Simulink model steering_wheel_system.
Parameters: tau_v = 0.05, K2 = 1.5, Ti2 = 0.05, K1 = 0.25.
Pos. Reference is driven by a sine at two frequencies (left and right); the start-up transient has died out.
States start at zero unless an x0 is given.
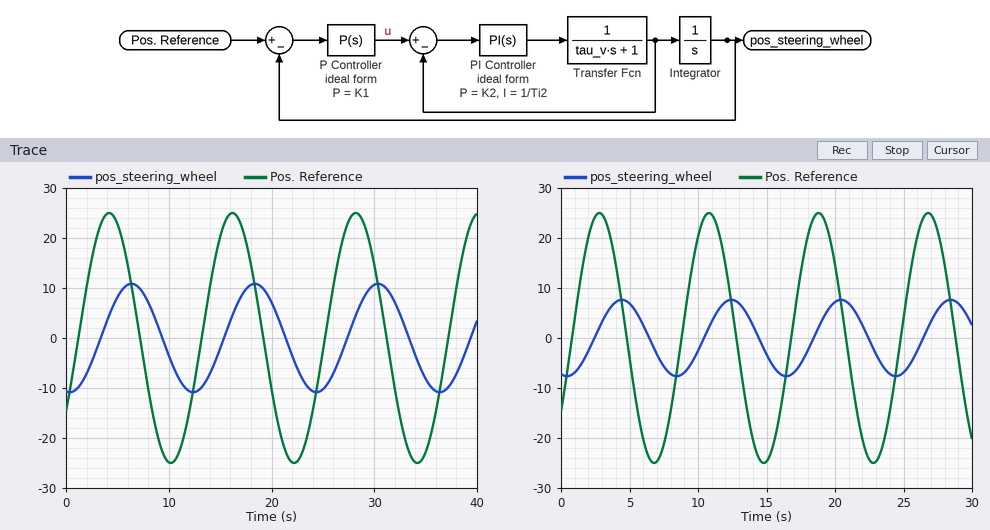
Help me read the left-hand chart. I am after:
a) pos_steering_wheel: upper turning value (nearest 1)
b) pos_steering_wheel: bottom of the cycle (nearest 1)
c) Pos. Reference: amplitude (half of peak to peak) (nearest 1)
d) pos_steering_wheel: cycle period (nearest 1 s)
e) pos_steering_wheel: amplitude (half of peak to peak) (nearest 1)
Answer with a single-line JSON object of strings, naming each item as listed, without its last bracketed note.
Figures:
{"pos_steering_wheel: upper turning value": "11", "pos_steering_wheel: bottom of the cycle": "-11", "Pos. Reference: amplitude (half of peak to peak)": "25", "pos_steering_wheel: cycle period": "12 s", "pos_steering_wheel: amplitude (half of peak to peak)": "11"}
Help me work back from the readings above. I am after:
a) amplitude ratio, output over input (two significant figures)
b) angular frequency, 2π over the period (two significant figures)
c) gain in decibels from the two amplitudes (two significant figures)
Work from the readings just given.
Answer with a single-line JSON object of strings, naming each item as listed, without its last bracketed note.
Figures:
{"amplitude ratio, output over input": "0.44", "angular frequency, 2π over the period": "0.52 rad/s", "gain in decibels from the two amplitudes": "-7.1 dB"}
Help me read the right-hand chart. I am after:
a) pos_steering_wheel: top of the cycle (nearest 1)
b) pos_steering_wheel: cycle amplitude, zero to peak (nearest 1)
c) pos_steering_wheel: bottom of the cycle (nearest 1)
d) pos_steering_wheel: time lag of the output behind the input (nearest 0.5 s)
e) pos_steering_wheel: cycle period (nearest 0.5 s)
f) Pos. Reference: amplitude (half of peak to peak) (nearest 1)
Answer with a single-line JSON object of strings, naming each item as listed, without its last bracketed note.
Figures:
{"pos_steering_wheel: top of the cycle": "8", "pos_steering_wheel: cycle amplitude, zero to peak": "8", "pos_steering_wheel: bottom of the cycle": "-8", "pos_steering_wheel: time lag of the output behind the input": "1.5 s", "pos_steering_wheel: cycle period": "8.0 s", "Pos. Reference: amplitude (half of peak to peak)": "25"}
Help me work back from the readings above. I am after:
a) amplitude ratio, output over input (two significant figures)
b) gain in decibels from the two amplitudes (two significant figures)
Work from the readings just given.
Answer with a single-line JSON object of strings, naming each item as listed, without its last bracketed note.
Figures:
{"amplitude ratio, output over input": "0.32", "gain in decibels from the two amplitudes": "-9.9 dB"}
